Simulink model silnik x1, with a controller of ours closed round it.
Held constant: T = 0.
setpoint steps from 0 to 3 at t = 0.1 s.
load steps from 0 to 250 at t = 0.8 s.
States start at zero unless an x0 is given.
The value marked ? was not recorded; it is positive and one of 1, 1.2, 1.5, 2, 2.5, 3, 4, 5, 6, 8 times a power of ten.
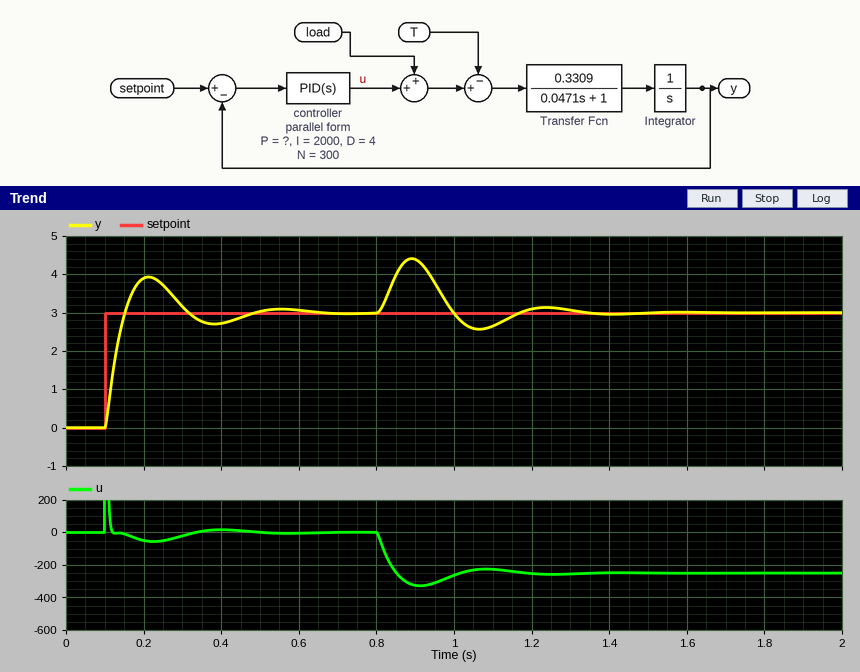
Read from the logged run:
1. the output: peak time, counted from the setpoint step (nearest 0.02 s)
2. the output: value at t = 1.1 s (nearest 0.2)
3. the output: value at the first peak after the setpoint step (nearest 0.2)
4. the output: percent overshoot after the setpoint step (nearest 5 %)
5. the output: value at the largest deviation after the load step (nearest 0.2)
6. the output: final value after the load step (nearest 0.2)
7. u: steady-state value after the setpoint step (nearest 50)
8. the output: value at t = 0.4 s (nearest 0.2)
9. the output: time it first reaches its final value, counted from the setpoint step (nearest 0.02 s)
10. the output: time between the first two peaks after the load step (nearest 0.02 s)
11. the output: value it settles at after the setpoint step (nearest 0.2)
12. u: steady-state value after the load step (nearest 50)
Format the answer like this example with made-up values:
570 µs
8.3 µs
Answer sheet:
0.12 s
2.6
4.0
30 %
4.4
3.0
0
2.8
0.06 s
0.34 s
3.0
-250
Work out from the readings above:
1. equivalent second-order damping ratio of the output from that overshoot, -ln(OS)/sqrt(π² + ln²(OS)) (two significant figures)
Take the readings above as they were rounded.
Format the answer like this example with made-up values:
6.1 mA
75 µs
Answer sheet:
0.36
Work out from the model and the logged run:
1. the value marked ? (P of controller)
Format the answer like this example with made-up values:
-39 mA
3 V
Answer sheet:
120
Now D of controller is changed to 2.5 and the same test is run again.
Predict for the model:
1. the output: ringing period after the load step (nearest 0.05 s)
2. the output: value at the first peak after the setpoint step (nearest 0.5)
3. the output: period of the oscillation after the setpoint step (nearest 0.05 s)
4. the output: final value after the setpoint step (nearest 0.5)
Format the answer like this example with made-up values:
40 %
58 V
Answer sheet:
0.30 s
4.5
0.30 s
3.0
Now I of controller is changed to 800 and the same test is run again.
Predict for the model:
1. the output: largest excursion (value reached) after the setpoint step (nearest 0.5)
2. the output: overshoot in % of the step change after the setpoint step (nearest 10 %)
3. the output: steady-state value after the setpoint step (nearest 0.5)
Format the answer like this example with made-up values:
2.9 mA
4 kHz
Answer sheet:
3.5
20 %
3.0
